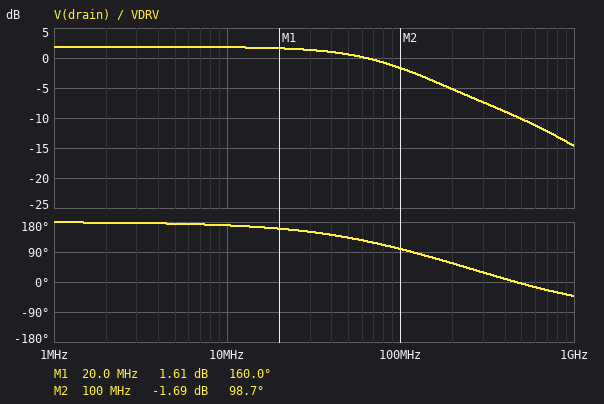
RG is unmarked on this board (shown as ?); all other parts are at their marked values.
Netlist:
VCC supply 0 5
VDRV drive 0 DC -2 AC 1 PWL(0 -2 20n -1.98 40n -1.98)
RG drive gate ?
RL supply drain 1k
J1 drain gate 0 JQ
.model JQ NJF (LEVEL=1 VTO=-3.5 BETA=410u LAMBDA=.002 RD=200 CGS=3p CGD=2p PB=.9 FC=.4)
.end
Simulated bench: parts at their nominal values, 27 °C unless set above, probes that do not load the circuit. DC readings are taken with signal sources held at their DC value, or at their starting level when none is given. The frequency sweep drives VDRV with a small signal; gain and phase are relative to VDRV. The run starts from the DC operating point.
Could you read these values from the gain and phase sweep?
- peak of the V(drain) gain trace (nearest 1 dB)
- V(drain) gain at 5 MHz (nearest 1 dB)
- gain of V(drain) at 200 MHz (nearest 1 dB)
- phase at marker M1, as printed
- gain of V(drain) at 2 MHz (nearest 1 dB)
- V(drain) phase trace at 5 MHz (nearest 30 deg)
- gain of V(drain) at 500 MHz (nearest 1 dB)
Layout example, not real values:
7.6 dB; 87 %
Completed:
2 dB; 2 dB; -5 dB; 160.0 deg; 2 dB; 180 deg; -10 dB
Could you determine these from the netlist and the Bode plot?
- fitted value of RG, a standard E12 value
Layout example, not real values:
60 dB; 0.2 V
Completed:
390 Ω
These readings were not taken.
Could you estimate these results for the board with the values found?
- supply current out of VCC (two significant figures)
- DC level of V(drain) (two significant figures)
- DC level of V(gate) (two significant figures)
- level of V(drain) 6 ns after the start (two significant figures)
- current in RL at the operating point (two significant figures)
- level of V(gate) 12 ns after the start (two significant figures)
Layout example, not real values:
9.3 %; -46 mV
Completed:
930 µA; 4.1 V; -2.0 V; 4.1 V; 930 µA; -2.0 V
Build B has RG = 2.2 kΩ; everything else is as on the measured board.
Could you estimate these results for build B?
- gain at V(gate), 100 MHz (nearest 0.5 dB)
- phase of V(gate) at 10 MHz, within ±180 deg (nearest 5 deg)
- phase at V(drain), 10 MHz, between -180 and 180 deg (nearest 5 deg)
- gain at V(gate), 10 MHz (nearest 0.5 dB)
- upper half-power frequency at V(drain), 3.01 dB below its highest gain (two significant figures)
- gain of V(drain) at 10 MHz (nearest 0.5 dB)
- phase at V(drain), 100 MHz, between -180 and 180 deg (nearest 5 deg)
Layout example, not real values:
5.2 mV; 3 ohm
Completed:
-13.5 dB; -25 deg; 150 deg; -1.0 dB; 20 MHz; 1.0 dB; 65 deg
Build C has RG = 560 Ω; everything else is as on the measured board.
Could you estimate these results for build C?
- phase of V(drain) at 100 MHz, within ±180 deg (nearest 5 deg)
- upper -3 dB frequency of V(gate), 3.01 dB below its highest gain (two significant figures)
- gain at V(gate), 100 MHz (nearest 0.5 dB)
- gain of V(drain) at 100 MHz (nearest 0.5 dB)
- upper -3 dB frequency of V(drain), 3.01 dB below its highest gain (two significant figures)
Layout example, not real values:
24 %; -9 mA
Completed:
90 deg; 72 MHz; -4.5 dB; -3.0 dB; 66 MHz
